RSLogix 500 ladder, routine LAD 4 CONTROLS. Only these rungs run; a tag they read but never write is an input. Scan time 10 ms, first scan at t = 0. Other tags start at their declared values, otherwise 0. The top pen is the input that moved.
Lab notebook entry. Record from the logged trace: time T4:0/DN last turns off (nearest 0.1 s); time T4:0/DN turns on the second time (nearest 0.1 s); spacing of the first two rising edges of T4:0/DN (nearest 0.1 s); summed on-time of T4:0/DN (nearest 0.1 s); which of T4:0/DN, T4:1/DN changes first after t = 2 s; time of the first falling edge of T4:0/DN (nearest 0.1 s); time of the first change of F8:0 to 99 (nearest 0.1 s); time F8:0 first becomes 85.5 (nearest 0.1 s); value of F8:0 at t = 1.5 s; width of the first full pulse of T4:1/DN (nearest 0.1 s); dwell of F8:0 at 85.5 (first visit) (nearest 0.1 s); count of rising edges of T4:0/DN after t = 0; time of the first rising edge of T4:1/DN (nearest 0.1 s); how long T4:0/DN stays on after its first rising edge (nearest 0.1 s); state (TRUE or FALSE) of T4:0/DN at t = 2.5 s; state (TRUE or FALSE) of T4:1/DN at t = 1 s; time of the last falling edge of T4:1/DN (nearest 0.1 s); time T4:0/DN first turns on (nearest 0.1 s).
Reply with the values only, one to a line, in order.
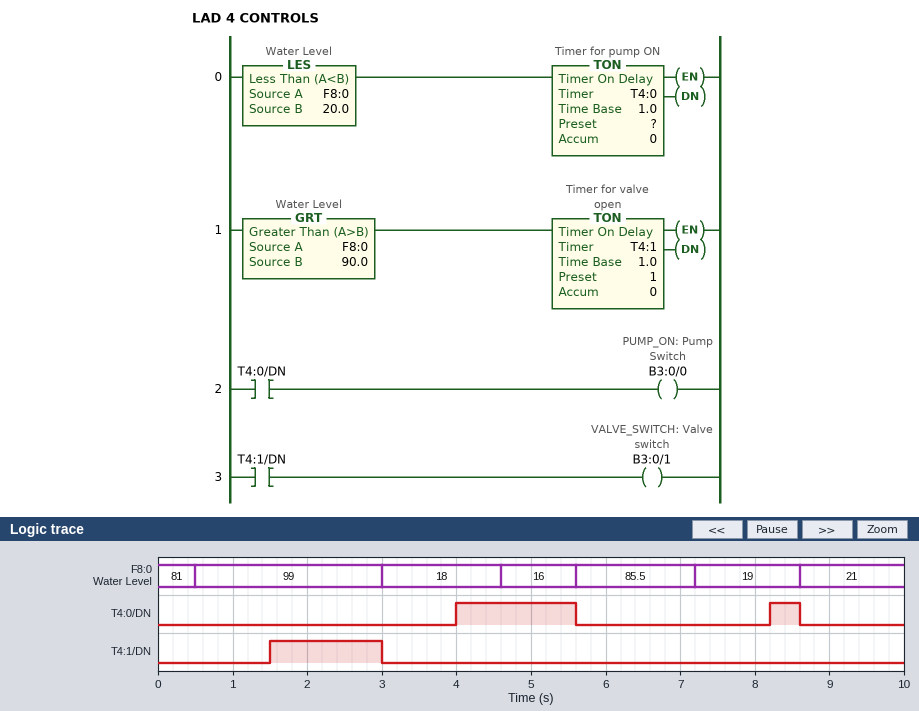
8.6 s
8.2 s
4.2 s
2.0 s
T4:1/DN
5.6 s
0.5 s
5.6 s
99
1.5 s
1.6 s
2
1.5 s
1.6 s
FALSE
FALSE
3.0 s
4.0 s
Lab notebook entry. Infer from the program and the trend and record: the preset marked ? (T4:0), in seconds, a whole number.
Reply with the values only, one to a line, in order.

1 s
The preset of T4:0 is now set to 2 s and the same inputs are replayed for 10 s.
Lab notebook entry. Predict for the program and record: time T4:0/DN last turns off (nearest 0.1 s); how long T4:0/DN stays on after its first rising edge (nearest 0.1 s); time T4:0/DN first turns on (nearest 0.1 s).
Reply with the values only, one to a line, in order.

5.6 s
0.6 s
5.0 s
